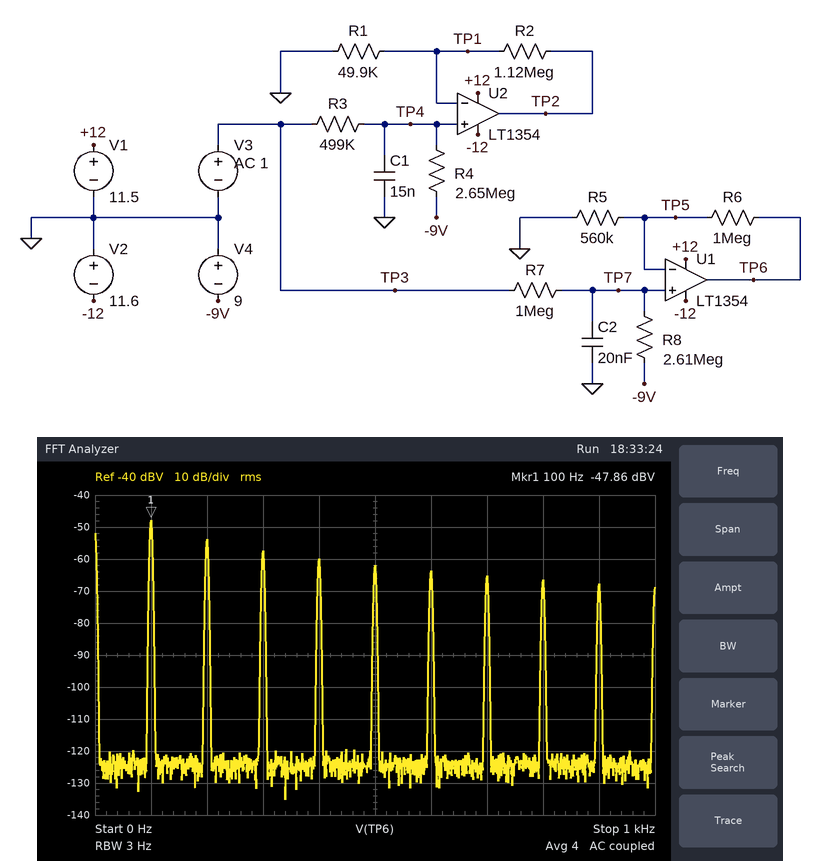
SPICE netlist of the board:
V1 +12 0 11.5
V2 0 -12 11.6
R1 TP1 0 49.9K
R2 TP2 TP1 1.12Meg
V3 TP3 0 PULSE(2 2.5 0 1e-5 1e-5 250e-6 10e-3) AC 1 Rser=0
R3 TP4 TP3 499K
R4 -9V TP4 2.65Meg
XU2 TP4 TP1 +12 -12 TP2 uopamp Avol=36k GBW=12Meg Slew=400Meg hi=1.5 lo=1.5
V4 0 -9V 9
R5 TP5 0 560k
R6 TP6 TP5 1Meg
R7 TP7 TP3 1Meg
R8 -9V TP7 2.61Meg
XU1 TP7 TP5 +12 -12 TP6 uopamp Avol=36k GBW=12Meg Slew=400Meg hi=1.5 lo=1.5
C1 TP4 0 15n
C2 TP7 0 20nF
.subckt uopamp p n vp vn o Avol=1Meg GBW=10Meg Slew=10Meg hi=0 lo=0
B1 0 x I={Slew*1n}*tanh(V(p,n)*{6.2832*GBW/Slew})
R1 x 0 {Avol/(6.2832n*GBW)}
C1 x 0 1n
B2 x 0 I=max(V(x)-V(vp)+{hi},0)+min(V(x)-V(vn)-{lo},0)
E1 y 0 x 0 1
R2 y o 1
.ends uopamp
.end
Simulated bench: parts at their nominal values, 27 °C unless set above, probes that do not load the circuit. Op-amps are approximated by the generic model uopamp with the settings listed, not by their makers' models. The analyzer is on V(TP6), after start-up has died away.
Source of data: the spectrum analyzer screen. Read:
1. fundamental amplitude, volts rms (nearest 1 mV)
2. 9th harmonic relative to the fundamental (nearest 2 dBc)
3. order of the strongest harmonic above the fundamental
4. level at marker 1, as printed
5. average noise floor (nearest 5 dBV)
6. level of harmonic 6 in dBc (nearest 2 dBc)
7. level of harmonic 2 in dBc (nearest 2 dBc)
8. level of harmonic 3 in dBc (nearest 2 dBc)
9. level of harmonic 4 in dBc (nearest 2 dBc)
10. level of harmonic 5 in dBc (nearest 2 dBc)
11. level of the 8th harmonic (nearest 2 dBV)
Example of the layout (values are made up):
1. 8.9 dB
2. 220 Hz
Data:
1. 4 mV
2. -20 dBc
3. 2
4. -47.86 dBV
5. -125 dBV
6. -16 dBc
7. -6 dBc
8. -10 dBc
9. -12 dBc
10. -14 dBc
11. -66 dBV
